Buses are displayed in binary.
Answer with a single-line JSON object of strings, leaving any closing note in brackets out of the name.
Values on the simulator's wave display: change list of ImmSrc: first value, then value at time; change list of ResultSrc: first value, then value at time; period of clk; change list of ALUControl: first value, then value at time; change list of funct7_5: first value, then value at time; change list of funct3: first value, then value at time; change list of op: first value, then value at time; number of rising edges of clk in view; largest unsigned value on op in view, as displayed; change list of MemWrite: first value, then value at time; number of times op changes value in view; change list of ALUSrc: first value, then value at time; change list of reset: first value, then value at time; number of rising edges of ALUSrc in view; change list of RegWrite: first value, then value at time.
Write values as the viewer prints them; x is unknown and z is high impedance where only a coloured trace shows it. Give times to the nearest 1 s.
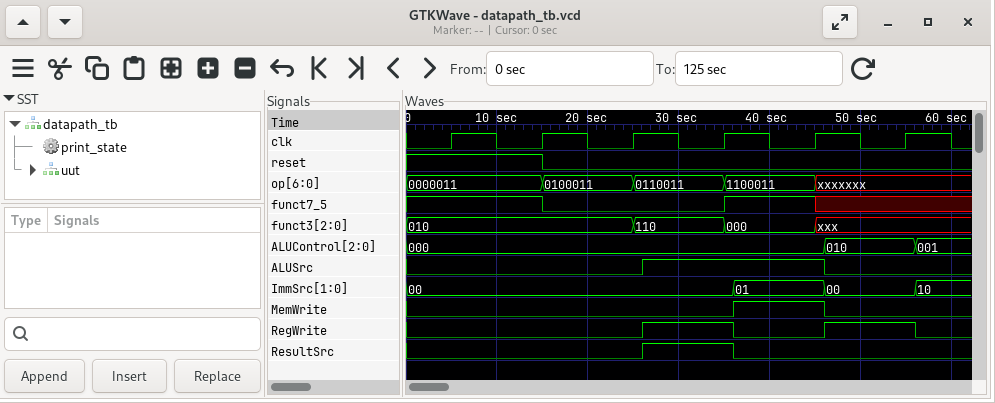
{"change list of ImmSrc: first value, then value at time": "00, 01 at 36 s, 00 at 46 s, 10 at 56 s", "change list of ResultSrc: first value, then value at time": "0, 1 at 26 s, 0 at 36 s", "period of clk": "10 s", "change list of ALUControl: first value, then value at time": "000, 010 at 46 s, 001 at 56 s", "change list of funct7_5: first value, then value at time": "1, 0 at 15 s, 1 at 35 s, x at 45 s", "change list of funct3: first value, then value at time": "010, 110 at 25 s, 000 at 35 s, xxx at 45 s", "change list of op: first value, then value at time": "0000011, 0100011 at 15 s, 0110011 at 25 s, 1100011 at 35 s, xxxxxxx at 45 s", "number of rising edges of clk in view": "6", "largest unsigned value on op in view, as displayed": "1100011", "change list of MemWrite: first value, then value at time": "0, 1 at 36 s, 0 at 46 s", "number of times op changes value in view": "4", "change list of ALUSrc: first value, then value at time": "0, 1 at 26 s, 0 at 46 s", "change list of reset: first value, then value at time": "1, 0 at 15 s", "number of rising edges of ALUSrc in view": "1", "change list of RegWrite: first value, then value at time": "0, 1 at 26 s, 0 at 36 s, 1 at 46 s, 0 at 56 s"}
